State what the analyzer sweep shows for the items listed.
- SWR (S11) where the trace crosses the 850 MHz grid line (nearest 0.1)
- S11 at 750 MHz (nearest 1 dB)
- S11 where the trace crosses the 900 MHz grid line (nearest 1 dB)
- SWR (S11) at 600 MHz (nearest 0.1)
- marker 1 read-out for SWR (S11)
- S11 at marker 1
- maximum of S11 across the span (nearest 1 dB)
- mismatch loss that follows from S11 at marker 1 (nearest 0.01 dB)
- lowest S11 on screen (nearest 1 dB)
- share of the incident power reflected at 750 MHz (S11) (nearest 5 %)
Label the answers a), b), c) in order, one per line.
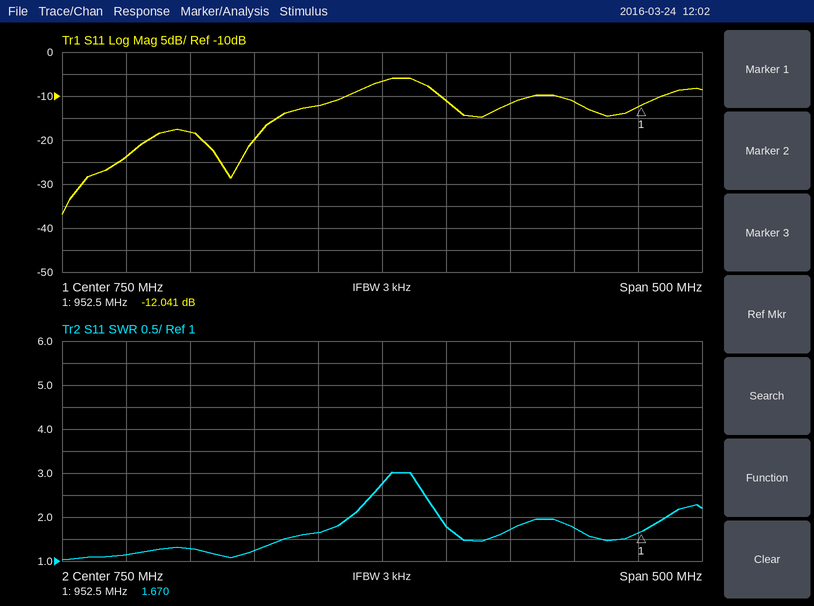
a) 1.7
b) -7 dB
c) -11 dB
d) 1.3
e) 1.670
f) -12.041 dB
g) -6 dB
h) 0.28 dB
i) -37 dB
j) 20 %
